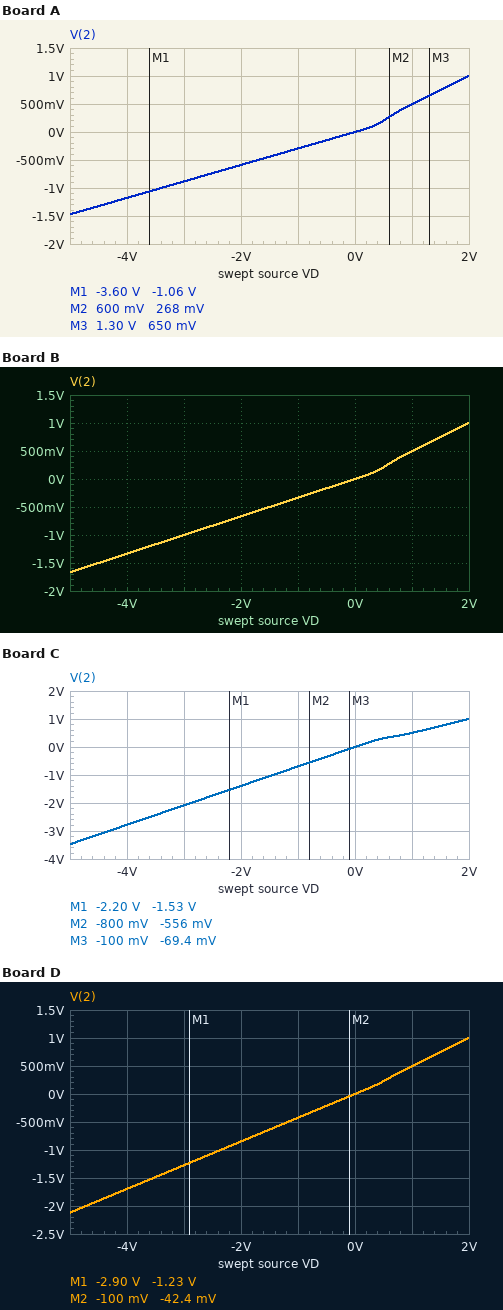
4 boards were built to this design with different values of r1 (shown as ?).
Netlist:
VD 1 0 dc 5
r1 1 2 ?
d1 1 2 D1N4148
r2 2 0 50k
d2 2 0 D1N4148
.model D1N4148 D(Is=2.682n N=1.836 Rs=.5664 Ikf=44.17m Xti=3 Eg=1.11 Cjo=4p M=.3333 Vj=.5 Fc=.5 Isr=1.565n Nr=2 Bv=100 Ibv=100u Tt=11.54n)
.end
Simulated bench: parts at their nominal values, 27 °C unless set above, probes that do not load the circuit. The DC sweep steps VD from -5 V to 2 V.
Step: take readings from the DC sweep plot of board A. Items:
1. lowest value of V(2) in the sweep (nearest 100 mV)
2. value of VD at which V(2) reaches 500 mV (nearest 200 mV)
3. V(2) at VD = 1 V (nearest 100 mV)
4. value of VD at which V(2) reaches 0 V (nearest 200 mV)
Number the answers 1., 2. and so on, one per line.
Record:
1. -1.5 V
2. 1.0 V
3. 500 mV
4. 0 V
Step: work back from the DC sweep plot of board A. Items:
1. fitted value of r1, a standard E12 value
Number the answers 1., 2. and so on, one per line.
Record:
1. 120 kΩ
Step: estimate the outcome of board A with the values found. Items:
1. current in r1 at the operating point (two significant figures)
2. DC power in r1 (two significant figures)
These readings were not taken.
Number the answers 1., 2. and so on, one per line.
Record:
1. 21 µA
2. 52 µW
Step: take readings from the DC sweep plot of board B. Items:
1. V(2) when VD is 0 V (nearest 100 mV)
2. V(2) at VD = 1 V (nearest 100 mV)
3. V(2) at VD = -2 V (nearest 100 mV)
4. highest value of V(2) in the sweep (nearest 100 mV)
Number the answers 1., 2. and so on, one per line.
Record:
1. 0 V
2. 500 mV
3. -700 mV
4. 1.0 V
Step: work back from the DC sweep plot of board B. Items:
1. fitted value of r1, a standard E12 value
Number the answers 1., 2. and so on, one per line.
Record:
1. 100 kΩ
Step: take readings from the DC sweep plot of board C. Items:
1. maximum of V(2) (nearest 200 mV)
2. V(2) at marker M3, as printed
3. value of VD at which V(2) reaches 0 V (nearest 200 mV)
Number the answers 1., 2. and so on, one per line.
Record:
1. 1.0 V
2. -69.4 mV
3. 0 V
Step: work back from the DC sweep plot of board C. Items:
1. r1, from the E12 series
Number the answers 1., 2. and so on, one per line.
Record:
1. 22 kΩ
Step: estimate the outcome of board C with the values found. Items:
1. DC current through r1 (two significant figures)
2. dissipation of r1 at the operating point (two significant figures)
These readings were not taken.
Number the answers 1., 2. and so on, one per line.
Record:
1. 110 µA
2. 280 µW
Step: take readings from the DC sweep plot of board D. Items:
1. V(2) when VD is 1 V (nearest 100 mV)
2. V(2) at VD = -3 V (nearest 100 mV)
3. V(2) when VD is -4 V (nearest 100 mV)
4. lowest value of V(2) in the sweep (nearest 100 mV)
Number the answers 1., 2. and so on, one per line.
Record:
1. 500 mV
2. -1.3 V
3. -1.7 V
4. -2.1 V
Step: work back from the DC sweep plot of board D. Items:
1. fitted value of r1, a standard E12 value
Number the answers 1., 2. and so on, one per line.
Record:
1. 68 kΩ
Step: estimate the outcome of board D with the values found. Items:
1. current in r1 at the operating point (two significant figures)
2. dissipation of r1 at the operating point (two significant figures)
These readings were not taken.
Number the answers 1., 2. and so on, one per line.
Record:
1. 37 µA
2. 92 µW
